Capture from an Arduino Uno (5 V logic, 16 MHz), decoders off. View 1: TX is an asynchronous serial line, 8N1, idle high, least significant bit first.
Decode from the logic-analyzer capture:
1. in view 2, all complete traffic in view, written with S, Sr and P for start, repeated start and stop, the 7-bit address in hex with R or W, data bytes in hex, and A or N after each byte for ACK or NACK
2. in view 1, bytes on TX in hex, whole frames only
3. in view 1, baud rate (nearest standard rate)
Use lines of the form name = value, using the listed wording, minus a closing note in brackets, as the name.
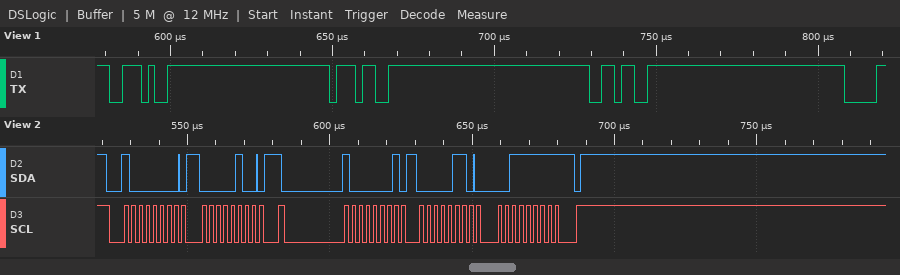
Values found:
in view 2, all complete traffic in view, written with S, Sr and P for start, repeated start and stop, the 7-bit address in hex with R or W, data bytes in hex, and A or N after each byte for ACK or NACK = S 40W A 04 A Sr 40R A 06 A 3F N P
in view 1, bytes on TX in hex, whole frames only = 2E 37 36
in view 1, baud rate = 500000 baud
